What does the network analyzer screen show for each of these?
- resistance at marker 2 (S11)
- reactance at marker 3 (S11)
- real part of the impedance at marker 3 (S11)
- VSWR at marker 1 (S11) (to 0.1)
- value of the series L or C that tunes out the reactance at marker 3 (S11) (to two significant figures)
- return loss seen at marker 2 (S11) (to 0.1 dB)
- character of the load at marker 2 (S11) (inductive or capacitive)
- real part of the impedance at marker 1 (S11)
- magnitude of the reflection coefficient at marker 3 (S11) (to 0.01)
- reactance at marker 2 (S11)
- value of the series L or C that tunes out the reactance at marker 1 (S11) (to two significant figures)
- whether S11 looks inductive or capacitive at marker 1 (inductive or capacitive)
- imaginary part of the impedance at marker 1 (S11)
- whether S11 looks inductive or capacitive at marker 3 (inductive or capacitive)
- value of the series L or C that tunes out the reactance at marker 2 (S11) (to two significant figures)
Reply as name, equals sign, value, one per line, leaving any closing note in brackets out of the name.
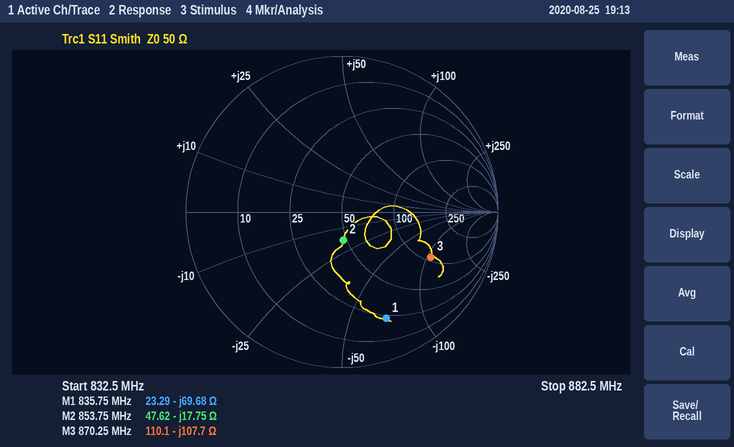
resistance at marker 2 = 47.62 Ω
reactance at marker 3 = -107.7 Ω
real part of the impedance at marker 3 = 110.1 Ω
VSWR at marker 1 (S11) = 6.6
value of the series L or C that tunes out the reactance at marker 3 (S11) = 20 nH
return loss seen at marker 2 (S11) = 14.9 dB
character of the load at marker 2 (S11) = capacitive
real part of the impedance at marker 1 = 23.29 Ω
magnitude of the reflection coefficient at marker 3 (S11) = 0.64
reactance at marker 2 = -17.75 Ω
value of the series L or C that tunes out the reactance at marker 1 (S11) = 13 nH
whether S11 looks inductive or capacitive at marker 1 = capacitive
imaginary part of the impedance at marker 1 = -69.68 Ω
whether S11 looks inductive or capacitive at marker 3 = capacitive
value of the series L or C that tunes out the reactance at marker 2 (S11) = 3.3 nH
